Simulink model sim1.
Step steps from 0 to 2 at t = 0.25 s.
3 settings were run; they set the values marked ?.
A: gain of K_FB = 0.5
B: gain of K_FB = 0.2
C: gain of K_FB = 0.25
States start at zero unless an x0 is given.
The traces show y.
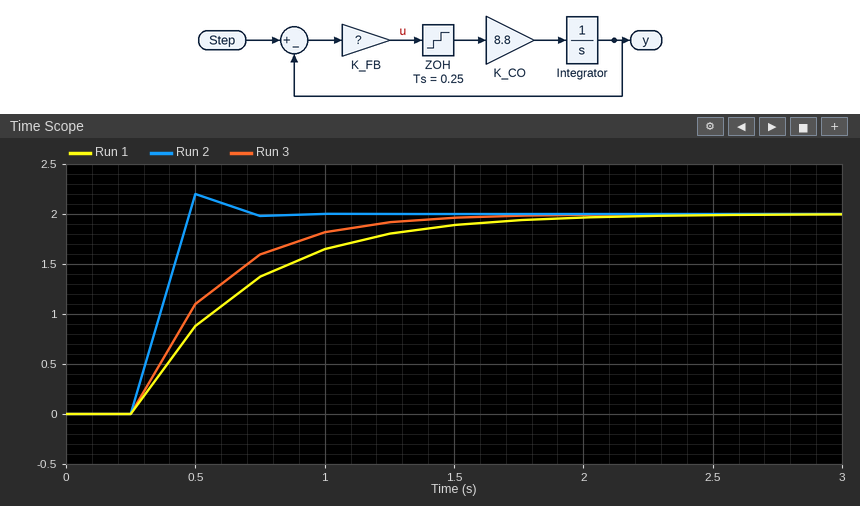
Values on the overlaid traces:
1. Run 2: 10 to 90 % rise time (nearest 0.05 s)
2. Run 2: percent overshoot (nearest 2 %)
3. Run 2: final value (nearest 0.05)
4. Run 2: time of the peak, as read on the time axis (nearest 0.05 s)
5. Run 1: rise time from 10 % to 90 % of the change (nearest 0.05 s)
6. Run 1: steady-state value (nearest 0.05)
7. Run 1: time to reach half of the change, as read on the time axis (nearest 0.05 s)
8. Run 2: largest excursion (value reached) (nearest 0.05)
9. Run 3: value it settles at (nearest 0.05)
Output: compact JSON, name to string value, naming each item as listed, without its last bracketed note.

{"Run 2: 10 to 90 % rise time": "0.20 s", "Run 2: percent overshoot": "10 %", "Run 2: final value": "2.00", "Run 2: time of the peak, as read on the time axis": "0.50 s", "Run 1: rise time from 10 % to 90 % of the change": "0.95 s", "Run 1: steady-state value": "2.00", "Run 1: time to reach half of the change, as read on the time axis": "0.55 s", "Run 2: largest excursion (value reached)": "2.20", "Run 3: value it settles at": "2.00"}
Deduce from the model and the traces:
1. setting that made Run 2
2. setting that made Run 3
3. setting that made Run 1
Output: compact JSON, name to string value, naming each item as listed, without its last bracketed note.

{"setting that made Run 2": "A", "setting that made Run 3": "C", "setting that made Run 1": "B"}
